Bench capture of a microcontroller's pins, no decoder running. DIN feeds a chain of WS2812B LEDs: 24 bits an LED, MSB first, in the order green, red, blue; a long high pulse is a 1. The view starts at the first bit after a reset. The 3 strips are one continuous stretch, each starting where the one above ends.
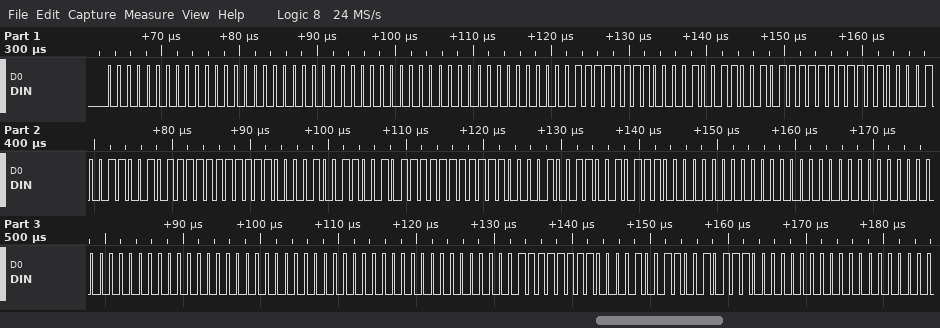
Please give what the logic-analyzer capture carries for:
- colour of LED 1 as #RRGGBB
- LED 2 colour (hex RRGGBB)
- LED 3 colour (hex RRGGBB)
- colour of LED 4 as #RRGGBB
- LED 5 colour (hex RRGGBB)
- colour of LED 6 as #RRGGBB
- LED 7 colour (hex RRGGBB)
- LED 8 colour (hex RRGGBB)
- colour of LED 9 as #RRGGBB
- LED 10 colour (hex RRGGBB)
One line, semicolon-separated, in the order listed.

#000000; #000000; #09FF97; #09FF97; #09FF97; #09FF97; #000000; #000000; #000000; #09FF97
